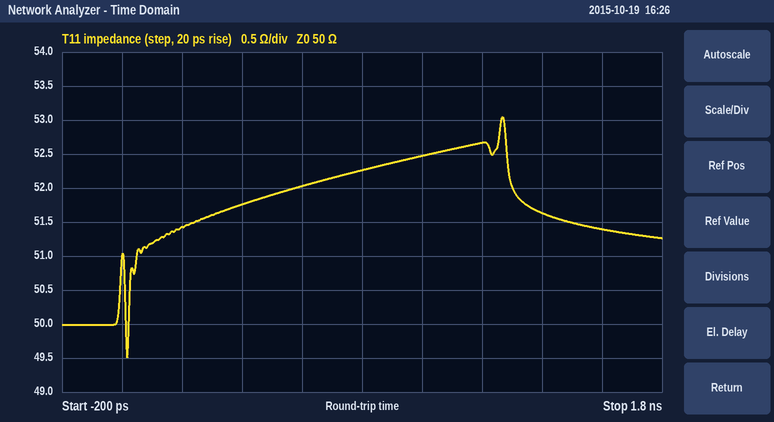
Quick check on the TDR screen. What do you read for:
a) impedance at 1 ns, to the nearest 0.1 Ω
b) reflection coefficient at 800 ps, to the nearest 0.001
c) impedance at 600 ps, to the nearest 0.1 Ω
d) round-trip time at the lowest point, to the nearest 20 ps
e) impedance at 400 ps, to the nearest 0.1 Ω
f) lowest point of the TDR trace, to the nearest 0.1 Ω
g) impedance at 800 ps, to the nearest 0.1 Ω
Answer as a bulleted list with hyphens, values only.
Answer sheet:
- 52.5 Ω
- +0.022
- 52.0 Ω
- 20 ps
- 51.8 Ω
- 49.5 Ω
- 52.3 Ω
